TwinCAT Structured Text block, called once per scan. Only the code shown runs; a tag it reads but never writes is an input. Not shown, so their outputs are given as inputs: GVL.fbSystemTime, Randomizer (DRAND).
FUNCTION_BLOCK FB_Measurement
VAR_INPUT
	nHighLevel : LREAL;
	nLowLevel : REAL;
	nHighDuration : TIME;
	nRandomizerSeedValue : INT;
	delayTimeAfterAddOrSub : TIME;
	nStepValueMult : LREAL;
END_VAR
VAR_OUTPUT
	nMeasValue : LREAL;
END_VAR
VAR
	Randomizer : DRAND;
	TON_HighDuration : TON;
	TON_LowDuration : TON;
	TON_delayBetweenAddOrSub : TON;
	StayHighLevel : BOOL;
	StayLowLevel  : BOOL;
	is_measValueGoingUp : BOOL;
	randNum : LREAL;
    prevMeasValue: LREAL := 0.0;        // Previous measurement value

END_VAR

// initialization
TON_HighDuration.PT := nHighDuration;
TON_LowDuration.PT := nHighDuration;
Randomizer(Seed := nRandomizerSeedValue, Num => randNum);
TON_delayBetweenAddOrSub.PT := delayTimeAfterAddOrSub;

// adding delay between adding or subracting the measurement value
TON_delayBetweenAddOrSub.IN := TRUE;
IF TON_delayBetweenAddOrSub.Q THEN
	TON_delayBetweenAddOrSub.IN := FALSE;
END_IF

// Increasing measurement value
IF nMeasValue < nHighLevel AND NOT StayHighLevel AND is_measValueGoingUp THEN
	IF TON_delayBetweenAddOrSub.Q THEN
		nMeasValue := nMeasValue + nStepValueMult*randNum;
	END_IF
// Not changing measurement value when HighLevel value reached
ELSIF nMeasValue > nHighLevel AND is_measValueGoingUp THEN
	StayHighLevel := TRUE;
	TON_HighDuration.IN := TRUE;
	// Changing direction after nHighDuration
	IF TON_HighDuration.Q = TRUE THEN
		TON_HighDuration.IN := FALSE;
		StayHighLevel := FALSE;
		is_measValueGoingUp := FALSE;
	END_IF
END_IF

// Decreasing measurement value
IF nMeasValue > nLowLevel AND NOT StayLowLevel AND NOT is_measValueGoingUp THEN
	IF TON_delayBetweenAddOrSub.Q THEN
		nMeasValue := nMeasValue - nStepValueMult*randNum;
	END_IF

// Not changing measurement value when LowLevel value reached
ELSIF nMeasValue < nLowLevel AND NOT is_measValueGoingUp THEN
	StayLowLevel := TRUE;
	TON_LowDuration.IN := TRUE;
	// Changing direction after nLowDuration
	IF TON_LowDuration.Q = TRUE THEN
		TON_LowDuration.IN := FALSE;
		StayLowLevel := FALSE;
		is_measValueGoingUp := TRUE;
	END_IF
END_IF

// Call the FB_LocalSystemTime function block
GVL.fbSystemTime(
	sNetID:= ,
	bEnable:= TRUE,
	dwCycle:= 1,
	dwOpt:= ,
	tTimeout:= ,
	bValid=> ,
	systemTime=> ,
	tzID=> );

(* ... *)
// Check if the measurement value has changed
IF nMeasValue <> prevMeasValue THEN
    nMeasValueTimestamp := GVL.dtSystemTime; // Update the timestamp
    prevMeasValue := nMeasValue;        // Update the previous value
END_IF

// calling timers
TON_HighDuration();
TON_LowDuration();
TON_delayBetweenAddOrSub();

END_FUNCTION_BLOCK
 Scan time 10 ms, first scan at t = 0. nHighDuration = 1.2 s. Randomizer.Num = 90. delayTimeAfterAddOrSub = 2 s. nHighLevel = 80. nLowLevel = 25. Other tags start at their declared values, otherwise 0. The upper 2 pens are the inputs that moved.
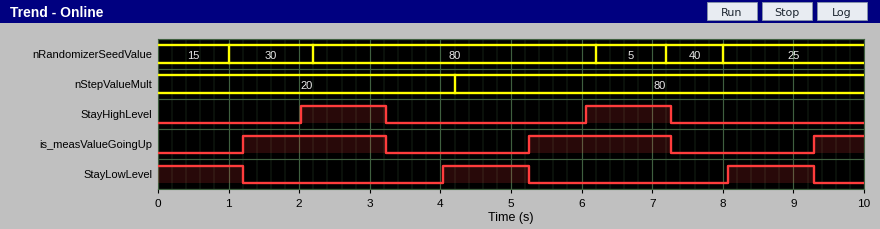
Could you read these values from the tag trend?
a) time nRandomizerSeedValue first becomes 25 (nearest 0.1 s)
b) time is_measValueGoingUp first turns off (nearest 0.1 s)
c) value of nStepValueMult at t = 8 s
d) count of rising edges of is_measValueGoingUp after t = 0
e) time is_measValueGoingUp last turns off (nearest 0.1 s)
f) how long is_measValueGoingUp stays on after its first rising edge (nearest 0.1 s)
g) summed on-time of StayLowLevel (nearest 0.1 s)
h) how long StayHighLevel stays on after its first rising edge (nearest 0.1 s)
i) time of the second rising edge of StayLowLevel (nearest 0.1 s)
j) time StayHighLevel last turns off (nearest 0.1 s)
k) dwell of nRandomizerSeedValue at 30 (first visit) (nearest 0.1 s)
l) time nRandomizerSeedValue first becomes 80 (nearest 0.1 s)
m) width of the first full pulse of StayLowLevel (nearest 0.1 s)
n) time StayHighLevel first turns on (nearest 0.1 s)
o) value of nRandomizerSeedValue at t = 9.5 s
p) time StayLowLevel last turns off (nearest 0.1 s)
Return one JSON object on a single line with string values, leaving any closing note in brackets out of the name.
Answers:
{"time nRandomizerSeedValue first becomes 25": "8.0 s", "time is_measValueGoingUp first turns off": "3.2 s", "value of nStepValueMult at t = 8 s": "80", "count of rising edges of is_measValueGoingUp after t = 0": "3", "time is_measValueGoingUp last turns off": "7.3 s", "how long is_measValueGoingUp stays on after its first rising edge": "2.0 s", "summed on-time of StayLowLevel": "3.6 s", "how long StayHighLevel stays on after its first rising edge": "1.2 s", "time of the second rising edge of StayLowLevel": "8.1 s", "time StayHighLevel last turns off": "7.3 s", "dwell of nRandomizerSeedValue at 30 (first visit)": "1.2 s", "time nRandomizerSeedValue first becomes 80": "2.2 s", "width of the first full pulse of StayLowLevel": "1.2 s", "time StayHighLevel first turns on": "2.0 s", "value of nRandomizerSeedValue at t = 9.5 s": "25", "time StayLowLevel last turns off": "9.3 s"}
